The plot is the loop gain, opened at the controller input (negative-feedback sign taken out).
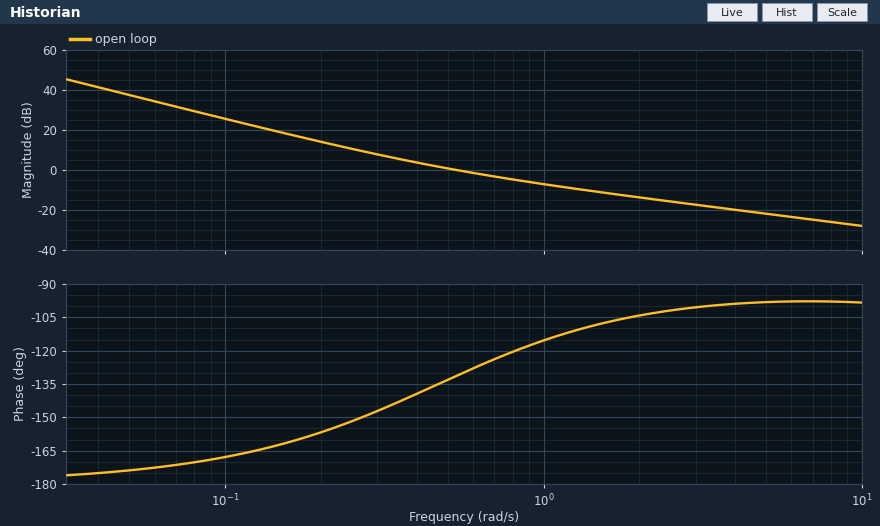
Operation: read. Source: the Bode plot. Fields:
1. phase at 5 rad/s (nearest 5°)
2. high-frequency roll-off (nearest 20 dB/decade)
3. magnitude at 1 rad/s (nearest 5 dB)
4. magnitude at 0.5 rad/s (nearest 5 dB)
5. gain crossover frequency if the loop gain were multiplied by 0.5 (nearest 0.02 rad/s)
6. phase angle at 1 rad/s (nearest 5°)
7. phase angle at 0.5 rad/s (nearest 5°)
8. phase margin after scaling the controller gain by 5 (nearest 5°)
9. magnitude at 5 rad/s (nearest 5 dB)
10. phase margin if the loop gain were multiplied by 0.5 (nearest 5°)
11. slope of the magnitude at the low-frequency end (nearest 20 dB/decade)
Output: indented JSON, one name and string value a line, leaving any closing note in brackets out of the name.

{
  "phase at 5 rad/s": "-100°",
  "high-frequency roll-off": "-20 dB/decade",
  "magnitude at 1 rad/s": "-5 dB",
  "magnitude at 0.5 rad/s": "0 dB",
  "gain crossover frequency if the loop gain were multiplied by 0.5": "0.34 rad/s",
  "phase angle at 1 rad/s": "-115°",
  "phase angle at 0.5 rad/s": "-135°",
  "phase margin after scaling the controller gain by 5": "75°",
  "magnitude at 5 rad/s": "-20 dB",
  "phase margin if the loop gain were multiplied by 0.5": "35°",
  "slope of the magnitude at the low-frequency end": "-40 dB/decade"
}
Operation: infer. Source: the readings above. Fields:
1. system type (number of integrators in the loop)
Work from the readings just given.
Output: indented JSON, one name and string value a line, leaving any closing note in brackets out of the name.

{
  "system type": "2"
}
